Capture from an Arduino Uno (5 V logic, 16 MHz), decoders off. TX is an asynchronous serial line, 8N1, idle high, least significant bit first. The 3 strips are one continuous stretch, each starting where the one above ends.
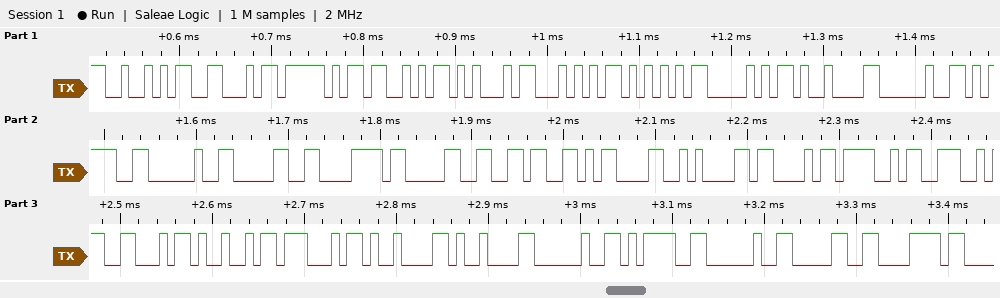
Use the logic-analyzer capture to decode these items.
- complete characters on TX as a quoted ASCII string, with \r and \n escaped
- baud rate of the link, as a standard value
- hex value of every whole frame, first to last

"RF_SETUP\t = 0x06\r\nCONFIG\t\t = 0x"
115200 baud
52 46 5F 53 45 54 55 50 09 20 3D 20 30 78 30 36 0D 0A 43 4F 4E 46 49 47 09 09 20 3D 20 30 78
